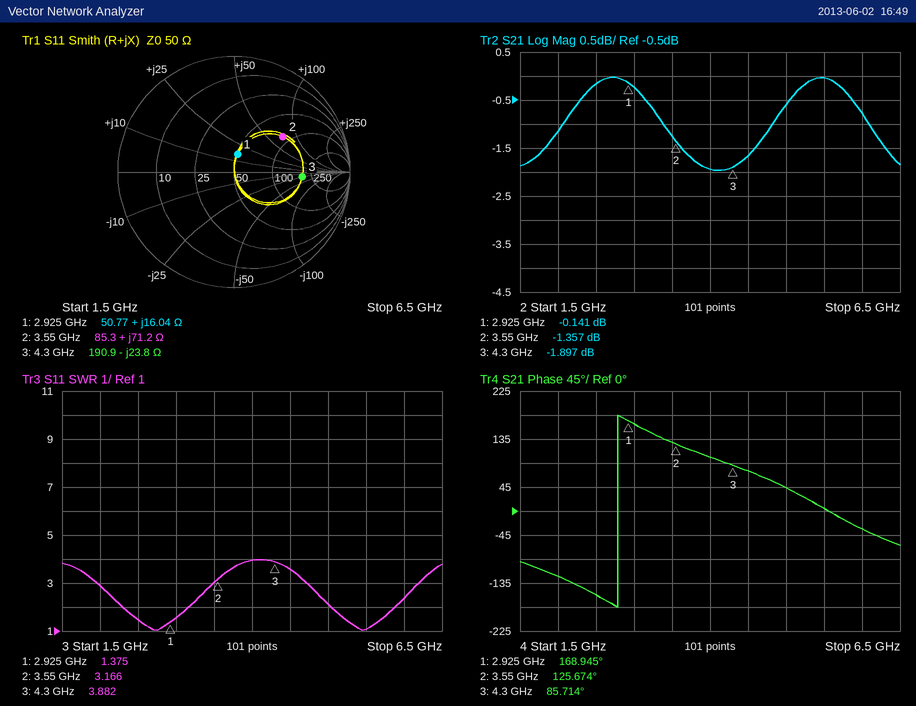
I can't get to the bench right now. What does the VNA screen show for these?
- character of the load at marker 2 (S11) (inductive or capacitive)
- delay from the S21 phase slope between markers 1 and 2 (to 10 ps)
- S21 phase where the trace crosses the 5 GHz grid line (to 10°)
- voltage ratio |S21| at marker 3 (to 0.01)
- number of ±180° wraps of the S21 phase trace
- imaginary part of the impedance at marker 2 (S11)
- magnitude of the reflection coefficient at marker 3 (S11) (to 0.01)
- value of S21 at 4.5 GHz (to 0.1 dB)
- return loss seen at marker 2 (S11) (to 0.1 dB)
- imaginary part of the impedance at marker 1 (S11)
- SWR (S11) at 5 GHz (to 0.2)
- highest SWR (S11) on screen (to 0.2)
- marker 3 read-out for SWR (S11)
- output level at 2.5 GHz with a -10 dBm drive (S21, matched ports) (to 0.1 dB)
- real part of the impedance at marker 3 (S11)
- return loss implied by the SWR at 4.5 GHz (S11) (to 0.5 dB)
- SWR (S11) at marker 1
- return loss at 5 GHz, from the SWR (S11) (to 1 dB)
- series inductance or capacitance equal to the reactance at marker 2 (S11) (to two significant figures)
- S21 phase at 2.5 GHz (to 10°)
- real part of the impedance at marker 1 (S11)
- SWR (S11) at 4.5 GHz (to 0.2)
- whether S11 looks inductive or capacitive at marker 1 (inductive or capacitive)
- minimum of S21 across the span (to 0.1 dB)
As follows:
inductive
190 ps
40°
0.80
1
+71.2 Ω
0.59
-1.7 dB
5.7 dB
+16.04 Ω
2.2
4.0
3.882
-10.2 dBm
190.9 Ω
5.0 dB
1.375
9 dB
3.2 nH
-160°
50.77 Ω
3.6
inductive
-2.0 dB
